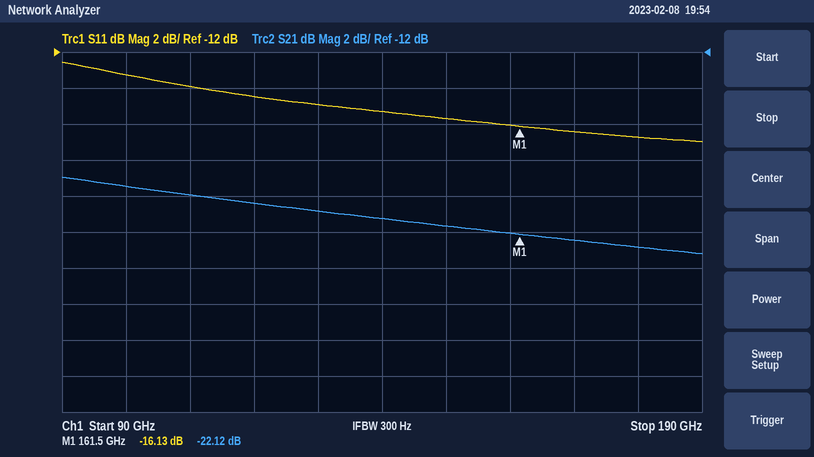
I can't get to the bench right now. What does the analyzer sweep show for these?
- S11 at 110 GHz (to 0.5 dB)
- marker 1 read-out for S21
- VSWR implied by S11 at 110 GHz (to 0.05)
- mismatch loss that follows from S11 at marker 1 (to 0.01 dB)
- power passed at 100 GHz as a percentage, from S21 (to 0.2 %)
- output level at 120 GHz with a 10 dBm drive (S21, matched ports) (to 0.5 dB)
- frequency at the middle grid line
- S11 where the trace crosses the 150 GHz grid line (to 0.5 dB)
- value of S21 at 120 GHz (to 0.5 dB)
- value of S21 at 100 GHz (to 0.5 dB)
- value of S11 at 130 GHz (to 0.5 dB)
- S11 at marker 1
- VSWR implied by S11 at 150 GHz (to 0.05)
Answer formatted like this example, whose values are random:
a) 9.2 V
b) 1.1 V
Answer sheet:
a) -14.0 dB
b) -22.12 dB
c) 1.50
d) 0.11 dB
e) 1.2 %
f) -10.5 dBm
g) 140 GHz
h) -15.5 dB
i) -20.5 dB
j) -19.5 dB
k) -15.0 dB
l) -16.13 dB
m) 1.40
